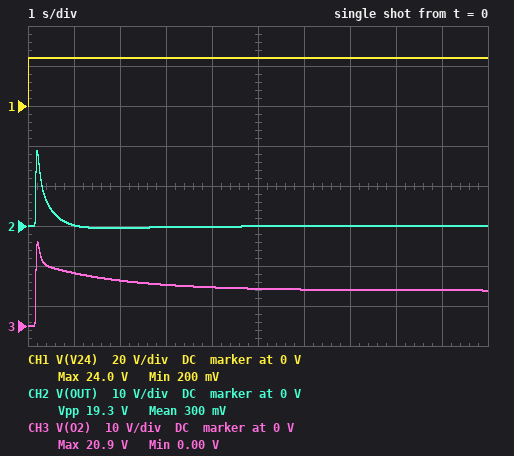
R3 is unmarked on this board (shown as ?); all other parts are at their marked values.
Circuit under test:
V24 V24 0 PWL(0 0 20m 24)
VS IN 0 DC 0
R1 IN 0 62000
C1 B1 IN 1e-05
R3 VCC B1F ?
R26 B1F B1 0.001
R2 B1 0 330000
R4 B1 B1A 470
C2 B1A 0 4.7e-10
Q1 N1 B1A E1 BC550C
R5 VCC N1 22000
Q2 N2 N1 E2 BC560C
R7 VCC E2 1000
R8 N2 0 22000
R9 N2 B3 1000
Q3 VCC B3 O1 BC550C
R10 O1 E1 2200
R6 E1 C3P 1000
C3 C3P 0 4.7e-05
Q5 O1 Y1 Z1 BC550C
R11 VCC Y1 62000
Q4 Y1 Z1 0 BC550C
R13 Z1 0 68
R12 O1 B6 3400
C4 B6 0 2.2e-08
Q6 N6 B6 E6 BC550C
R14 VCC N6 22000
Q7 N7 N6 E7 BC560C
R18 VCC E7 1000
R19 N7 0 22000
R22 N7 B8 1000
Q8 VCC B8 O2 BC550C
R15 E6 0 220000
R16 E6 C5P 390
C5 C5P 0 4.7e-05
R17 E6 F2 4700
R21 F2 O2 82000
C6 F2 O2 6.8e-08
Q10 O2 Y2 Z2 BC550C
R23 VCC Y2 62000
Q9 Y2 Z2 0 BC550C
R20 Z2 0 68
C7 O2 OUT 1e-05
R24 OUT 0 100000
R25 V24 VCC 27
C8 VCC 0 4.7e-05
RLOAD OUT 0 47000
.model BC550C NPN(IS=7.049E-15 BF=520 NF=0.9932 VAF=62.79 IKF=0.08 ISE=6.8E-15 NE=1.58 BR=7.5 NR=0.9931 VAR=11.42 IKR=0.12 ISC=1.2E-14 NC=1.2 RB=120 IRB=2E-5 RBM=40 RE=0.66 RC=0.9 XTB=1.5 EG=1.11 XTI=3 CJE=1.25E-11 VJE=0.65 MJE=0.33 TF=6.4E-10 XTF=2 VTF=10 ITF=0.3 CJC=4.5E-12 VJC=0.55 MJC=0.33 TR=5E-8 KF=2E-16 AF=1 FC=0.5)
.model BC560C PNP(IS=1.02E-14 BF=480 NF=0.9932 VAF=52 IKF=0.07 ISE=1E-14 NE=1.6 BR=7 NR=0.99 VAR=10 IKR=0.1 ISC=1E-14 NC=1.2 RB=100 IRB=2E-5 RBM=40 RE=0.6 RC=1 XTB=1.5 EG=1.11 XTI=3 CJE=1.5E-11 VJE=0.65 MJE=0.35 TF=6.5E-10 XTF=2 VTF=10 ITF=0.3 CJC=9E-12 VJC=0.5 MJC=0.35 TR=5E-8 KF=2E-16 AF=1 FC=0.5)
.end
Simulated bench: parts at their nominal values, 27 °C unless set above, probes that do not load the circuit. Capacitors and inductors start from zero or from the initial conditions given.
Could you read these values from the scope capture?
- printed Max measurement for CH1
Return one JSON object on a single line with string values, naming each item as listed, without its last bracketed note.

{"printed Max measurement for CH1": "24.0 V"}
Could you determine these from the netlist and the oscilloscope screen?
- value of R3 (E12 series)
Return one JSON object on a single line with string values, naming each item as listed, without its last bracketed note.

{"value of R3": "390 kΩ"}
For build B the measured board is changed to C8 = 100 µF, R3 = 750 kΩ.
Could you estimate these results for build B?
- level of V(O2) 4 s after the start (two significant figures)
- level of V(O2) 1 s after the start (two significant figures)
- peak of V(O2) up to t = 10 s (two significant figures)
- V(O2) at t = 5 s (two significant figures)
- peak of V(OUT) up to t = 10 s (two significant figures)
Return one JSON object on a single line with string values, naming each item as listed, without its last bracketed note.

{"level of V(O2) 4 s after the start": "5.1 V", "level of V(O2) 1 s after the start": "6.2 V", "peak of V(O2) up to t = 10 s": "6.7 V", "V(O2) at t = 5 s": "5.0 V", "peak of V(OUT) up to t = 10 s": "5.7 V"}
